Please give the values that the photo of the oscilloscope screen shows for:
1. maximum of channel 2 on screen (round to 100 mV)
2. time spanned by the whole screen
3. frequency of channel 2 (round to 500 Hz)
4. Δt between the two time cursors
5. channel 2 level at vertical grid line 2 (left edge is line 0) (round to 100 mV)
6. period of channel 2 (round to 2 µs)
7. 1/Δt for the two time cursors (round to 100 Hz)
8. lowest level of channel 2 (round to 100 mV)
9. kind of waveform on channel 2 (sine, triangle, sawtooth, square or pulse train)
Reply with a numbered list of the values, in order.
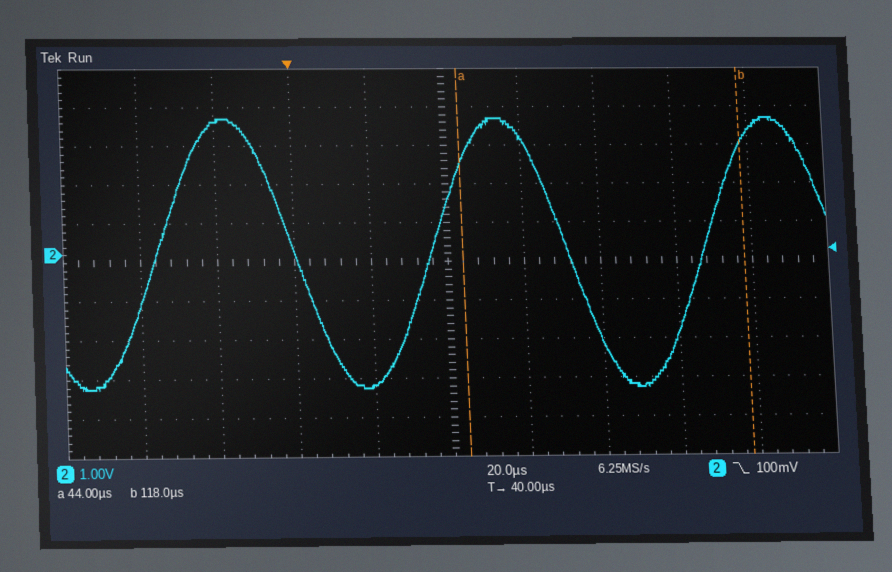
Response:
1. 3.5 V
2. 200 µs
3. 14.0 kHz
4. 74 µs
5. 3.4 V
6. 72 µs
7. 13.5 kHz
8. -3.4 V
9. sine
